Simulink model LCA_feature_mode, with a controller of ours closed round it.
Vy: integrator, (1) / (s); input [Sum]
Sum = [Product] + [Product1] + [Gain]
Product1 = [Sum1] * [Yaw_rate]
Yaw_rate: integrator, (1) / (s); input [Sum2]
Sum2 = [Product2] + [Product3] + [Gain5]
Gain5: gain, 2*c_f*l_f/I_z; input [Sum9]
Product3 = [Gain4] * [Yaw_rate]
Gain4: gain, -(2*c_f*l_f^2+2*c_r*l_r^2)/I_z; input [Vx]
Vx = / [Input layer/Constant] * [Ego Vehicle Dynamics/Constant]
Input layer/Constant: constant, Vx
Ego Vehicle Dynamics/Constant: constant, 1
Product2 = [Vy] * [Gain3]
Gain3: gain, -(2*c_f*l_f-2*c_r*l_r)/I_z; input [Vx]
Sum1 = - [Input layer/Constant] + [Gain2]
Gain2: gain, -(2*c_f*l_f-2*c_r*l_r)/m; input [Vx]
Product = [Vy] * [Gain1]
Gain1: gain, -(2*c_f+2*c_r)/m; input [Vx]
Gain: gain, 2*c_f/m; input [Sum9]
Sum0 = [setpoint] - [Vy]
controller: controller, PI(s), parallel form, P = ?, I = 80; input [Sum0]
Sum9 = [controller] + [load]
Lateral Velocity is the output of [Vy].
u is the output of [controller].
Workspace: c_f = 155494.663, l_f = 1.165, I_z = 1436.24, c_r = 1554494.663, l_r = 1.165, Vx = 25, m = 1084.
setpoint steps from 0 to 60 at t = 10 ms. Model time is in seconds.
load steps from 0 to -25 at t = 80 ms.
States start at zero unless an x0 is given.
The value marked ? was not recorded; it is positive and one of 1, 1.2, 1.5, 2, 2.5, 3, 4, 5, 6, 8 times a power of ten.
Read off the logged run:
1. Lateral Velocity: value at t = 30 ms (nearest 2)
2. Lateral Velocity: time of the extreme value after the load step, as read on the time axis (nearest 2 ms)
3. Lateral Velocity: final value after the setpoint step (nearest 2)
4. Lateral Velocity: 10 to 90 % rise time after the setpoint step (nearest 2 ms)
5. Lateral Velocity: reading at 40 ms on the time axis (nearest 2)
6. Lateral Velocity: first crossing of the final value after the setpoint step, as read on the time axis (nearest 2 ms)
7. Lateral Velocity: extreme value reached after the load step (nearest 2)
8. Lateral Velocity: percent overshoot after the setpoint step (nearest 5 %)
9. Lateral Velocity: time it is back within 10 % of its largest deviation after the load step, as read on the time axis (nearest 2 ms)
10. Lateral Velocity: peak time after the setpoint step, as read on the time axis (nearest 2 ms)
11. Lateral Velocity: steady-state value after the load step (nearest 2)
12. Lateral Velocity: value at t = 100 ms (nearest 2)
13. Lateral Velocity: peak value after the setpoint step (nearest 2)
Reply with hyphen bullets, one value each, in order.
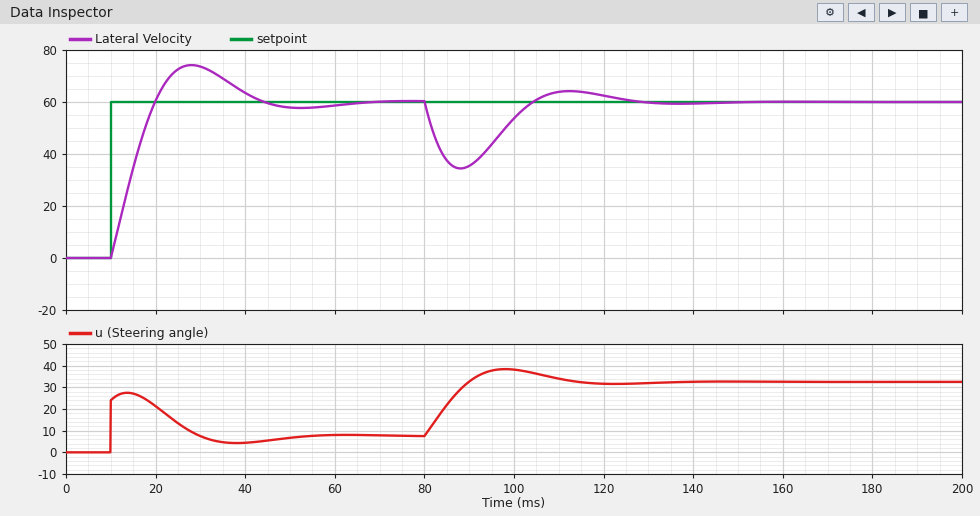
- 74
- 88 ms
- 60
- 8 ms
- 64
- 20 ms
- 34
- 25 %
- 120 ms
- 28 ms
- 60
- 54
- 74
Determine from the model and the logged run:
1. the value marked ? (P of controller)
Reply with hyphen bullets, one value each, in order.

- 0.4
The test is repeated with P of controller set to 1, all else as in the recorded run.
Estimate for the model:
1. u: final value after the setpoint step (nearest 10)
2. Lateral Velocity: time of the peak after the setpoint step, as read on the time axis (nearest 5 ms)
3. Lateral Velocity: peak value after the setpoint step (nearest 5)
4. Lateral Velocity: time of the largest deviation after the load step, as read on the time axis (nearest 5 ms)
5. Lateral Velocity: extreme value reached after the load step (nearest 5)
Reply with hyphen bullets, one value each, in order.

- 10
- 25 ms
- 65
- 85 ms
- 45
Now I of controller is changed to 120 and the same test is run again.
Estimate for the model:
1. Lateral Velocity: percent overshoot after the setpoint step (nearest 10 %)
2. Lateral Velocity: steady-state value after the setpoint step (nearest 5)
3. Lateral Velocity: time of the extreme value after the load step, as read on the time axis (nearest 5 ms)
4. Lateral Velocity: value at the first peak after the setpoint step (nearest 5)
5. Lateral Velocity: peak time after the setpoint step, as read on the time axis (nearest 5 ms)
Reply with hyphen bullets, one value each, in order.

- 30 %
- 60
- 85 ms
- 80
- 25 ms
